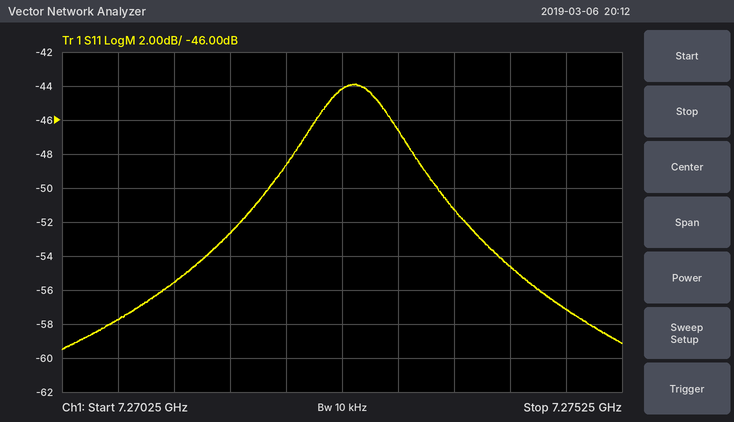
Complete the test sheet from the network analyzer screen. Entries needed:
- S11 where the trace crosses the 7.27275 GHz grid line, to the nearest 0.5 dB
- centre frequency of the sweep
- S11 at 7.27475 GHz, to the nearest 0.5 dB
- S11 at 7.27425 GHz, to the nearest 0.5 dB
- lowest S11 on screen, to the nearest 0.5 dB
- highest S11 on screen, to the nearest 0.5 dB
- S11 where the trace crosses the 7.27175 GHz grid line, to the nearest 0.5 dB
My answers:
-44.0 dB
7.27275 GHz
-57.0 dB
-54.5 dB
-59.5 dB
-44.0 dB
-52.5 dB
